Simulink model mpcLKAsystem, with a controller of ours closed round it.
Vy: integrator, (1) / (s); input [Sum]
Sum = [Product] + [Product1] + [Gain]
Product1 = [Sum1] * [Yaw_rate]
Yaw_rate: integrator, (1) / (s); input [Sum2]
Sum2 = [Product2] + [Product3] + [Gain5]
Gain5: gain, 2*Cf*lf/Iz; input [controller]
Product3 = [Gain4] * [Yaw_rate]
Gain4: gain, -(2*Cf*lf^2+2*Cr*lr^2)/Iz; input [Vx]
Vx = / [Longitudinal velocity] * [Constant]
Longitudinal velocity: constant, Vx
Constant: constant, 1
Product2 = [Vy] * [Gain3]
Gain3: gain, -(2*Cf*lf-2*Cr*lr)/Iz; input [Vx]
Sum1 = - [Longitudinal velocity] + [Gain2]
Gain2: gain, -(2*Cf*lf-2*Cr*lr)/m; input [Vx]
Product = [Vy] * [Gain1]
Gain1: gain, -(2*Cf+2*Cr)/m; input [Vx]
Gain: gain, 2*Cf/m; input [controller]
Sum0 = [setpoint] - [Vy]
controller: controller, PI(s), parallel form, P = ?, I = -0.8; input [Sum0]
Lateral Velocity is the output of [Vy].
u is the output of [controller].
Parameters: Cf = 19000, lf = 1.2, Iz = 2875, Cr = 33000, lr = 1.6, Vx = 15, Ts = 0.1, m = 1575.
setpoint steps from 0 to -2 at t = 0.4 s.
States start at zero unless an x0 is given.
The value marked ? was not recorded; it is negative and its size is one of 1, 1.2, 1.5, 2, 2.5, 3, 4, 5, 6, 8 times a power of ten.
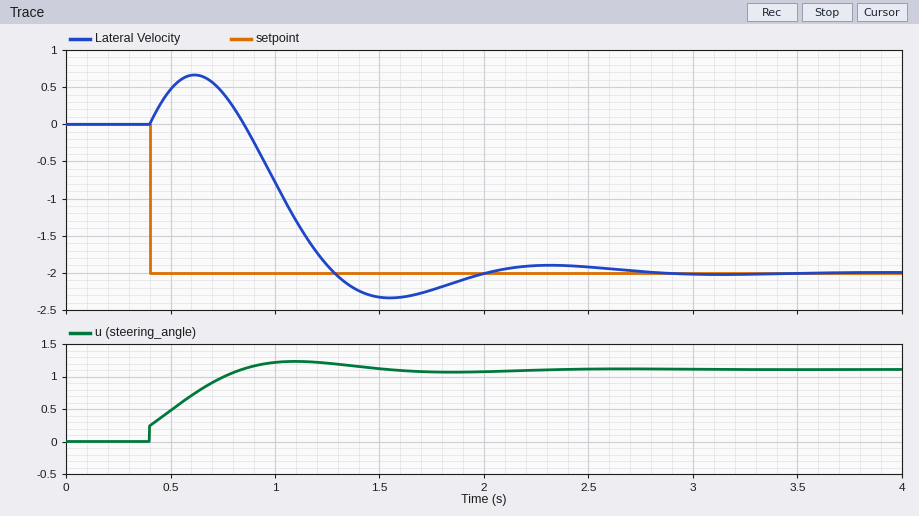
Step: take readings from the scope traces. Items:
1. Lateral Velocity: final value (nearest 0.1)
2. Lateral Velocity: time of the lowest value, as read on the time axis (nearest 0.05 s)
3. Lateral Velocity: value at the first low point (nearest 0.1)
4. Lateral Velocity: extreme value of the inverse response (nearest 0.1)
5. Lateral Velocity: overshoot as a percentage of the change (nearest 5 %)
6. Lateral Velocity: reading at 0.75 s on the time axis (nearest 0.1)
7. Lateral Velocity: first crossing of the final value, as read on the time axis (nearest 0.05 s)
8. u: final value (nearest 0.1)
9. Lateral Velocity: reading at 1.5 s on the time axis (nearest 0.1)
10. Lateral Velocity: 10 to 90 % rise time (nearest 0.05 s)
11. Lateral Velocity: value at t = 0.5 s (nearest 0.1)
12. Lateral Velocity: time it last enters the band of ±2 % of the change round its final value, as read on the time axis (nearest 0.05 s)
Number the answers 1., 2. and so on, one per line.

1. -2.0
2. 1.55 s
3. -2.3
4. 0.7
5. 15 %
6. 0.4
7. 1.30 s
8. 1.1
9. -2.3
10. 0.35 s
11. 0.5
12. 2.65 s
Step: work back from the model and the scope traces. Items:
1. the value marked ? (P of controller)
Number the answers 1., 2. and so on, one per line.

1. -0.12
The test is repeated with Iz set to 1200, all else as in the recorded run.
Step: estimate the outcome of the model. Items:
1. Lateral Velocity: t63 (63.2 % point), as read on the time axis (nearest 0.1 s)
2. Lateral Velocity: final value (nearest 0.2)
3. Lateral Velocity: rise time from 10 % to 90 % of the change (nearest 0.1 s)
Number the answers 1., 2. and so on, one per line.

1. 1.0 s
2. -2.0
3. 1.1 s
